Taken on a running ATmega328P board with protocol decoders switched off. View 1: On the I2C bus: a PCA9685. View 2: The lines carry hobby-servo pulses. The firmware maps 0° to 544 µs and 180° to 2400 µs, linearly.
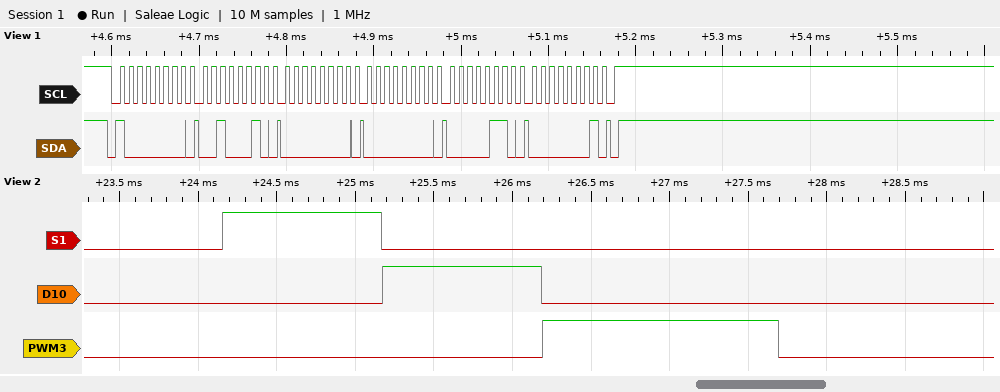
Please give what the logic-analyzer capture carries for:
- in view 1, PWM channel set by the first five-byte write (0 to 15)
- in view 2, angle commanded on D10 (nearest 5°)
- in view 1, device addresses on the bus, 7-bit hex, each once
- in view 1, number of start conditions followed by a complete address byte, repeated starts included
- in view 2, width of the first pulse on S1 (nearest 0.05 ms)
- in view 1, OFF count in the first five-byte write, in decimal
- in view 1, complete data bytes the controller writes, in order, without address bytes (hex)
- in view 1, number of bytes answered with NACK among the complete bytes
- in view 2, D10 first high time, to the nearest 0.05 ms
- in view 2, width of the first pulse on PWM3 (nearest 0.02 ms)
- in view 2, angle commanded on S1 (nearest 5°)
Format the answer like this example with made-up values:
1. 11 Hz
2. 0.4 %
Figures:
1. 7
2. 45°
3. 0x40
4. 1
5. 1.00 ms
6. 262
7. 22 00 00 06 01
8. 0
9. 1.00 ms
10. 1.50 ms
11. 45°
